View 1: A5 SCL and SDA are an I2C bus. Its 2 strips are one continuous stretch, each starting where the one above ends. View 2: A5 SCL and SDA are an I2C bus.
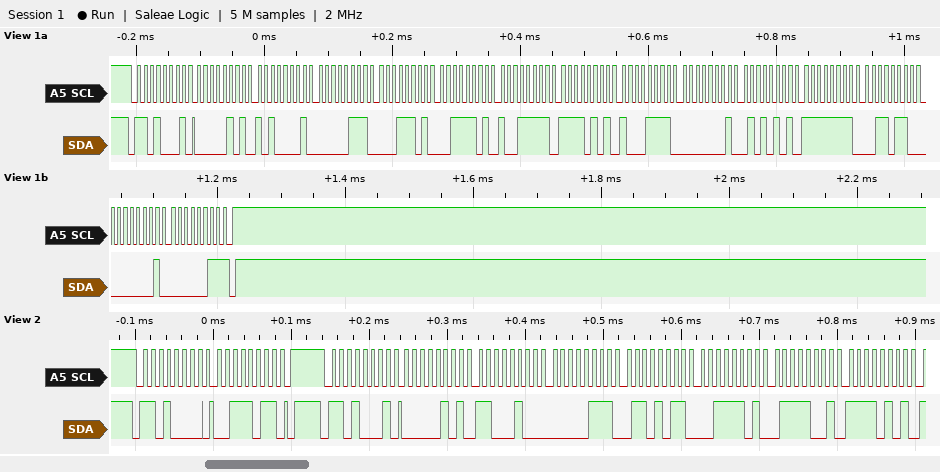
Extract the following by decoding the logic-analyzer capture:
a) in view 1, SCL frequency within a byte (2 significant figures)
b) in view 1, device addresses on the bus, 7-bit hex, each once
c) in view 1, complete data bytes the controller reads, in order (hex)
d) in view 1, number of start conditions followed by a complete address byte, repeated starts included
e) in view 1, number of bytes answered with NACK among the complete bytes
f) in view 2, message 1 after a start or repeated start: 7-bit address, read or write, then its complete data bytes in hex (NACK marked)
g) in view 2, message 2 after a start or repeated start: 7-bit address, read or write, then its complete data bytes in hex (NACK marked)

100 kHz
0x68
05 A1 07 1D 3D 9F F5 8F 01 55 FF 36 01 03
1
1
0x68 write: 3B
0x68 read: 05 C4 07 6B 3D 79 F5
